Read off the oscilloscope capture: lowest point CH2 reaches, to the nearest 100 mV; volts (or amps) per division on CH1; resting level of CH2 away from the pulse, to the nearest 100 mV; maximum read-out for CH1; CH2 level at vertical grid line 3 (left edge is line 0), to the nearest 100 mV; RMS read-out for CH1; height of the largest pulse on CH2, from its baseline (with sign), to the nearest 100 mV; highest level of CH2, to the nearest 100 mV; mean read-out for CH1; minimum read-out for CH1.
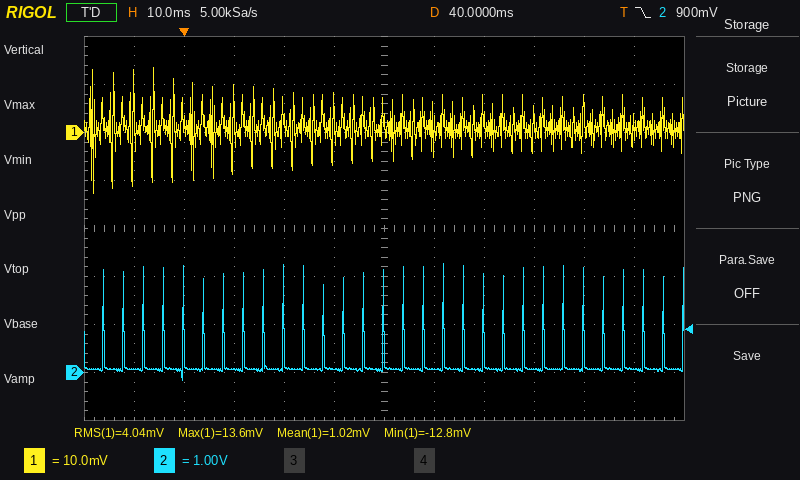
-200 mV
10 mV
100 mV
13.6 mV
100 mV
4.04 mV
+2.2 V
2.3 V
1.02 mV
-12.8 mV
